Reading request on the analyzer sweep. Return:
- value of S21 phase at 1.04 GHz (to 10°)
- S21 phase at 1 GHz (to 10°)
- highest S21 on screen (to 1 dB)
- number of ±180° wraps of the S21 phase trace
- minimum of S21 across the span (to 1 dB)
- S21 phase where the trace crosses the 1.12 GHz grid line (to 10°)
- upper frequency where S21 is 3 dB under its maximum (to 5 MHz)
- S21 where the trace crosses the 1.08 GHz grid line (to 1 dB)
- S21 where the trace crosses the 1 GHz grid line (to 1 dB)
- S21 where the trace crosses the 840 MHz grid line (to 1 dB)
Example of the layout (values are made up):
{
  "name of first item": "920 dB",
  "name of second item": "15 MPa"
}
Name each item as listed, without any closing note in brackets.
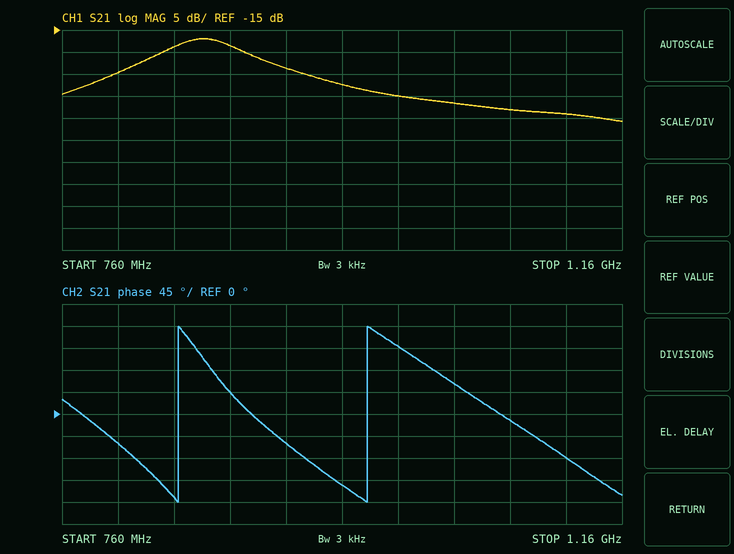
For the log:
{
  "value of S21 phase at 1.04 GHz": "60°",
  "S21 phase at 1 GHz": "140°",
  "highest S21 on screen": "-17 dB",
  "number of ±180° wraps of the S21 phase trace": "2",
  "minimum of S21 across the span": "-36 dB",
  "S21 phase where the trace crosses the 1.12 GHz grid line": "-90°",
  "upper frequency where S21 is 3 dB under its maximum": "890 MHz",
  "S21 where the trace crosses the 1.08 GHz grid line": "-33 dB",
  "S21 where the trace crosses the 1 GHz grid line": "-30 dB",
  "S21 where the trace crosses the 840 MHz grid line": "-19 dB"
}
